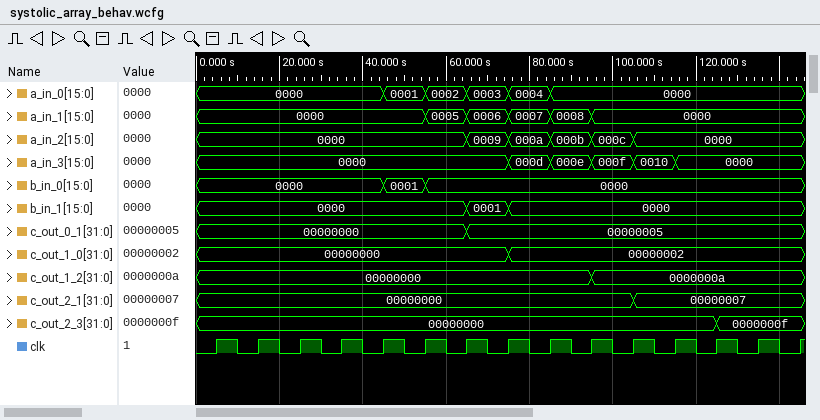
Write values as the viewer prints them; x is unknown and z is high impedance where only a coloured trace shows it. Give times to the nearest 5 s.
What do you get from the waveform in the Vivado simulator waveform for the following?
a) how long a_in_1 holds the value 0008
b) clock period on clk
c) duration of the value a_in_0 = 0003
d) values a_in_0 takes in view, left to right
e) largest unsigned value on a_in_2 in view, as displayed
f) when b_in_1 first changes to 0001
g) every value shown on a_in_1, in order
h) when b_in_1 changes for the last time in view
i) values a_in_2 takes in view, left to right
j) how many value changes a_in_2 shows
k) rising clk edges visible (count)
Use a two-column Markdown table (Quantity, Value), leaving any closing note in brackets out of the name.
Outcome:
| Quantity | Value |
|---|---|
| how long a_in_1 holds the value 0008 | 10 s |
| clock period on clk | 10 s |
| duration of the value a_in_0 = 0003 | 10 s |
| values a_in_0 takes in view, left to right | 0000, 0001, 0002, 0003, 0004, 0000 |
| largest unsigned value on a_in_2 in view, as displayed | 000c |
| when b_in_1 first changes to 0001 | 65 s |
| every value shown on a_in_1, in order | 0000, 0005, 0006, 0007, 0008, 0000 |
| when b_in_1 changes for the last time in view | 75 s |
| values a_in_2 takes in view, left to right | 0000, 0009, 000a, 000b, 000c, 0000 |
| how many value changes a_in_2 shows | 5 |
| rising clk edges visible | 15 |
